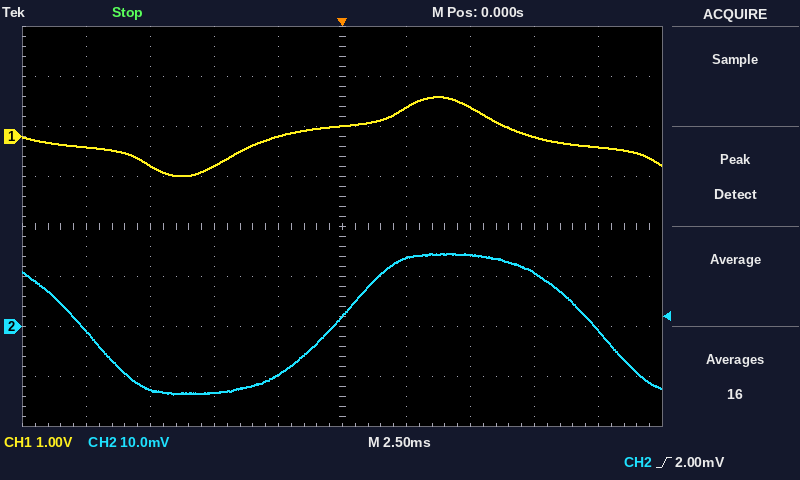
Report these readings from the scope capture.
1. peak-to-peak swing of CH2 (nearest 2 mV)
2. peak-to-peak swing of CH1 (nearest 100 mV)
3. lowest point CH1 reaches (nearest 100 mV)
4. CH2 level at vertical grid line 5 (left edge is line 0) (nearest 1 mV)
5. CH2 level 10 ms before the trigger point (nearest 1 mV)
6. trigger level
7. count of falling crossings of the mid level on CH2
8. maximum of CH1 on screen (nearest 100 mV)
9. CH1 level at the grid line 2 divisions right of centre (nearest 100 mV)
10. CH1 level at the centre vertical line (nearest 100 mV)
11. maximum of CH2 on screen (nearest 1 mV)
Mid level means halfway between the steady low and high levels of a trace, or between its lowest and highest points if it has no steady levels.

28 mV
1.6 V
-800 mV
2 mV
-1 mV
2.00 mV
2
800 mV
600 mV
200 mV
15 mV
